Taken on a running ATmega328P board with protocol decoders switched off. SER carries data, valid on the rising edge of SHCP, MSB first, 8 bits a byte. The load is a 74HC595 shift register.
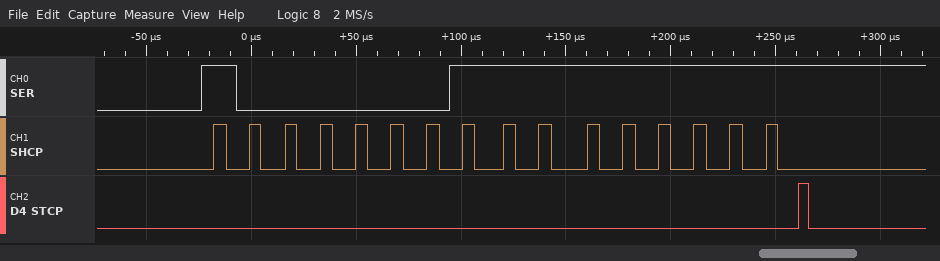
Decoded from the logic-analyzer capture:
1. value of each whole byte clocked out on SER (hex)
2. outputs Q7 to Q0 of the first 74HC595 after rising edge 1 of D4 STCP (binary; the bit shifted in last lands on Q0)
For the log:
81 FF
11111111
